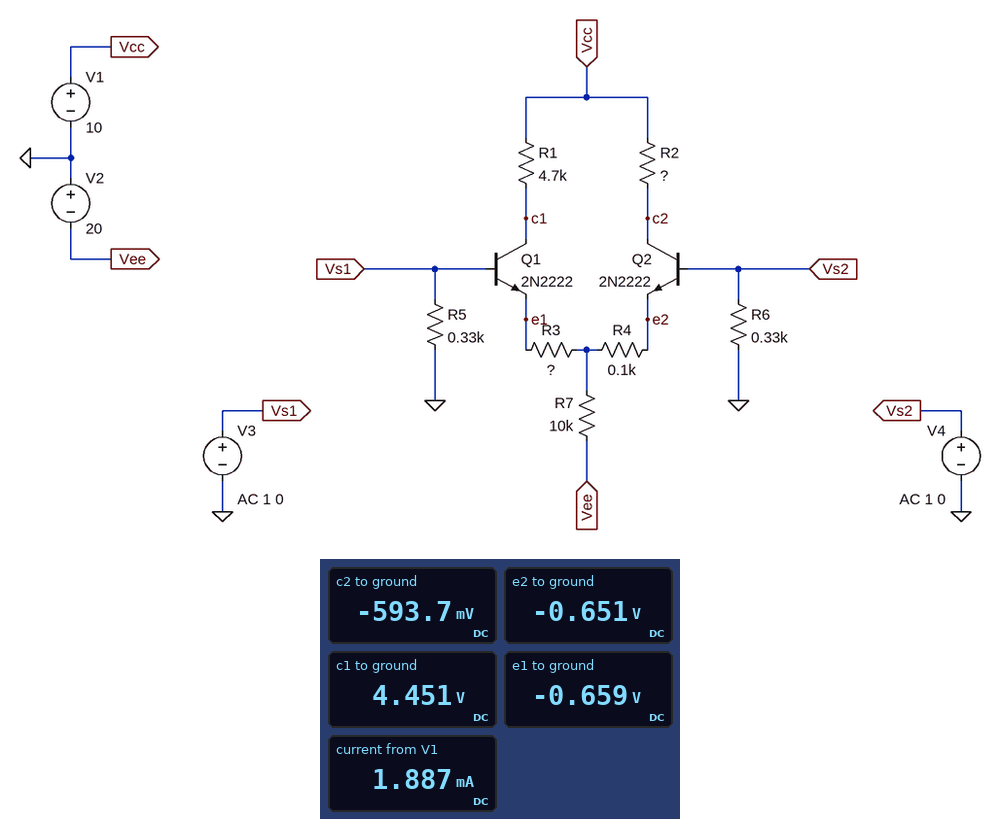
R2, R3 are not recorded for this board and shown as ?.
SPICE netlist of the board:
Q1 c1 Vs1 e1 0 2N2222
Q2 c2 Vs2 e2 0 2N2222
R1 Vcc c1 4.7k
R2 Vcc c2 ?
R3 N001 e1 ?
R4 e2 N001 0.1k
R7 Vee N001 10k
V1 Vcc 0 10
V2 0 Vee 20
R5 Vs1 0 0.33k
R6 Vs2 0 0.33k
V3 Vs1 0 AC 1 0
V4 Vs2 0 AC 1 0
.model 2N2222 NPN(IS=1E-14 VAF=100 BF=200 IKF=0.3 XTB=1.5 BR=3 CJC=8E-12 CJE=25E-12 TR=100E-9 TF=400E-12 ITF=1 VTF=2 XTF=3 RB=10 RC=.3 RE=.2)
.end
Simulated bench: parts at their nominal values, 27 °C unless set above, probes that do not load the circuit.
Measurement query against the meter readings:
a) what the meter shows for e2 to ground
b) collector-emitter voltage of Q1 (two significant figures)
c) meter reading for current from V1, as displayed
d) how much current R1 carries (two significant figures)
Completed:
-0.651 V
5.1 V
1.887 mA
1.2 mA
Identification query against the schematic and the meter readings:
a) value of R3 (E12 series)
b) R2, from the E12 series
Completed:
56 Ω
15 kΩ
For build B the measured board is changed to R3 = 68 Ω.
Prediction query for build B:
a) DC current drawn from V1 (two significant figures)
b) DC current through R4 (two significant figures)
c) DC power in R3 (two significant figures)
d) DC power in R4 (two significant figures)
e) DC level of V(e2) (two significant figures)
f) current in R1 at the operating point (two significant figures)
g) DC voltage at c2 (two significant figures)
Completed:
1.8 mA
790 µA
88 µW
62 µW
-660 mV
1.1 mA
-620 mV
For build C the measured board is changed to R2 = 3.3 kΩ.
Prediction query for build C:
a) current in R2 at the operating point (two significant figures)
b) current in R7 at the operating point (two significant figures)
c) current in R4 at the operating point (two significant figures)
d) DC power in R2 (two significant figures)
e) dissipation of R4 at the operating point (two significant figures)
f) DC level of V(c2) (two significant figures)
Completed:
760 µA
1.9 mA
770 µA
1.9 mW
59 µW
7.5 V
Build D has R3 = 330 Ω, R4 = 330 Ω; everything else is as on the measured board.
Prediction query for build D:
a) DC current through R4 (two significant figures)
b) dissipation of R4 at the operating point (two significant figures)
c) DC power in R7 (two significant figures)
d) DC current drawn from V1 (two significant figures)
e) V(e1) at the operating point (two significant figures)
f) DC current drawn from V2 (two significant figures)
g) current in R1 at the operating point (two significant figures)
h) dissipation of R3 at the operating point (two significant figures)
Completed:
930 µA
280 µW
36 mW
1.7 mA
-650 mV
1.9 mA
970 µA
310 µW
